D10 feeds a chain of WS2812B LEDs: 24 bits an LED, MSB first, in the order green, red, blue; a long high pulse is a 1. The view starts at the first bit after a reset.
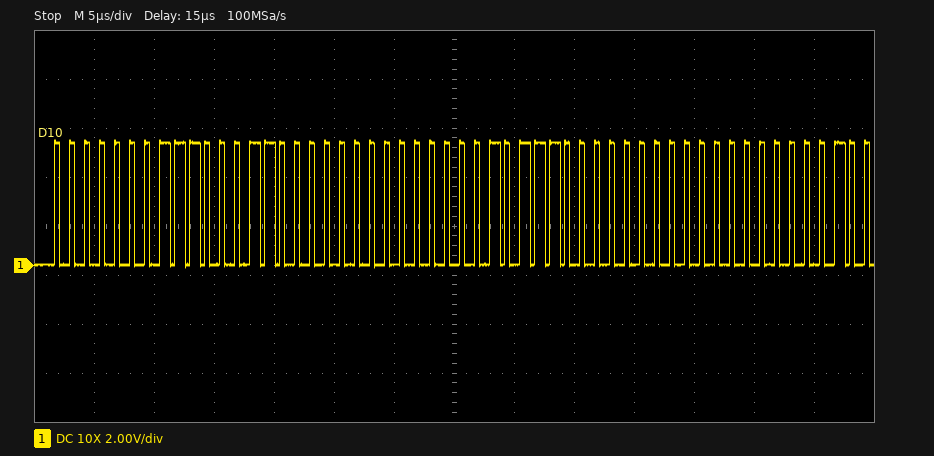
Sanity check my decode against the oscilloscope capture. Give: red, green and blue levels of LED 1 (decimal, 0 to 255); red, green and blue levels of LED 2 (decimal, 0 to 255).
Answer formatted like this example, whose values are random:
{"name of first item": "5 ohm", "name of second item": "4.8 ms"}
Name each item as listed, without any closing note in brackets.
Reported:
{"red, green and blue levels of LED 1": "198, 1, 0", "red, green and blue levels of LED 2": "192, 5, 0"}
